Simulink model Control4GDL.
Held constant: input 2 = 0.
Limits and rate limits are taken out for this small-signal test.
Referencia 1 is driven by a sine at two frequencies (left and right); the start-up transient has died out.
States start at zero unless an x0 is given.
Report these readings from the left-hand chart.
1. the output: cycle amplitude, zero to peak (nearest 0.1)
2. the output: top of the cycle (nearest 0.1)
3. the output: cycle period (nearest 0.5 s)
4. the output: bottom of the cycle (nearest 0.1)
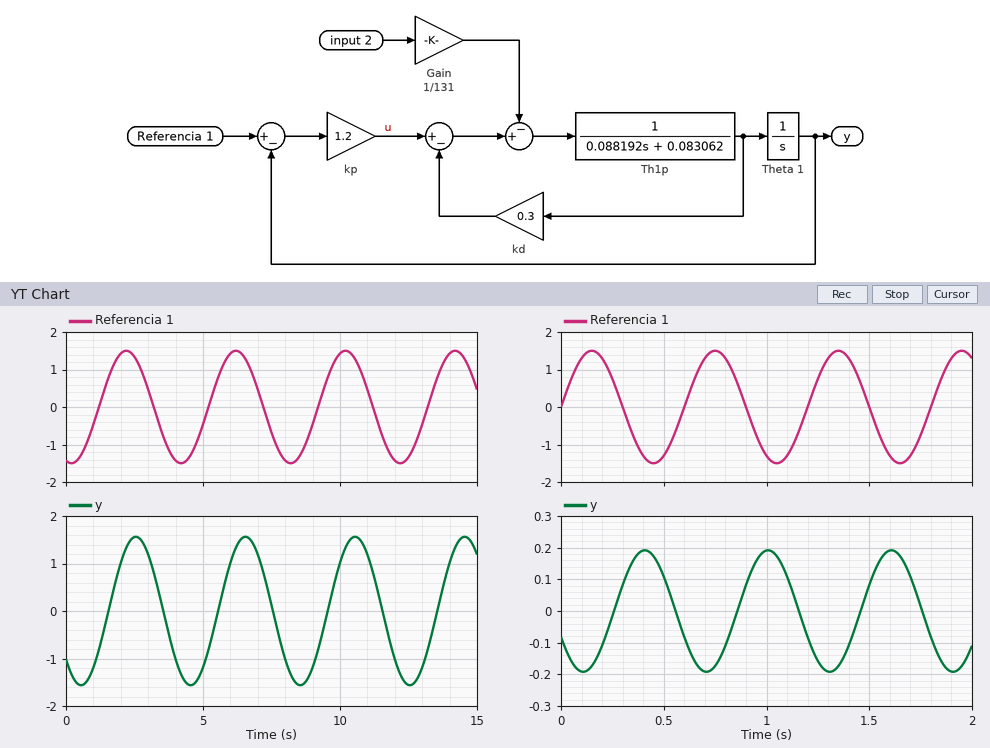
1.6
1.6
4.0 s
-1.6
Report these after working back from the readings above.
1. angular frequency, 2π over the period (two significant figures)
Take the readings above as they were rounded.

1.6 rad/s
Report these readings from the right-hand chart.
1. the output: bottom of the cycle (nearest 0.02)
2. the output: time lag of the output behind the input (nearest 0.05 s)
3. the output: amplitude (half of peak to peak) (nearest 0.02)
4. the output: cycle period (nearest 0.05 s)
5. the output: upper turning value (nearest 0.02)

-0.20
0.25 s
0.20
0.60 s
0.20
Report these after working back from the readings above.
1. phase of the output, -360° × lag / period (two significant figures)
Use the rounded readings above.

-150°
